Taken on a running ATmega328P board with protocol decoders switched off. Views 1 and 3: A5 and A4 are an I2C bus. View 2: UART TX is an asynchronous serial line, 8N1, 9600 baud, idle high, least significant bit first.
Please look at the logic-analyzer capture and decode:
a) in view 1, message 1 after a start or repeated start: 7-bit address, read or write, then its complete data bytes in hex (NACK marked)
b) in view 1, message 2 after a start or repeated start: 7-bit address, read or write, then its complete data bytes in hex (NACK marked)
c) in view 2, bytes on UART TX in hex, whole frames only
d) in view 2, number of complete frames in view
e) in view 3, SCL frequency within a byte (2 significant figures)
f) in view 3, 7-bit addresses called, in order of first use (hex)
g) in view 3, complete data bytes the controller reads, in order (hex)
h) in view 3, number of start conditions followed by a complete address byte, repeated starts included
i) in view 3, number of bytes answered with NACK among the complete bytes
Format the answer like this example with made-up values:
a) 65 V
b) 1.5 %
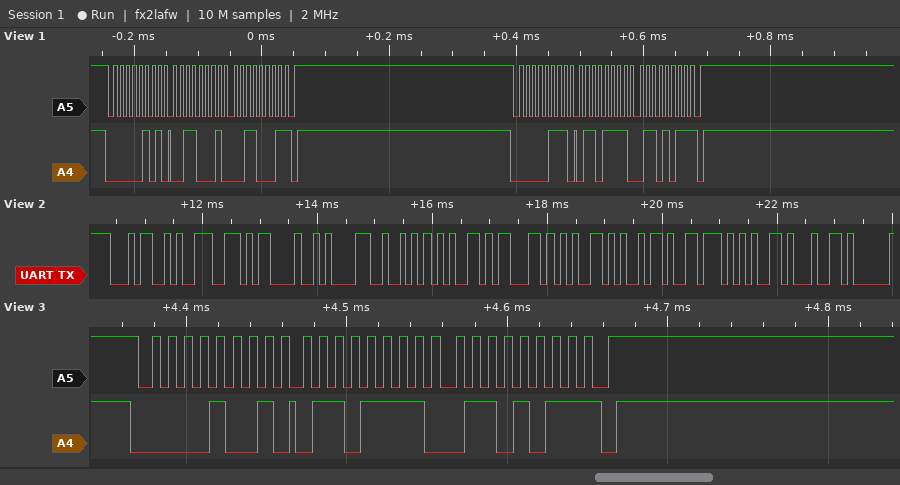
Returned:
a) 0x02 read: 31 31 NACK
b) 0x03 read: 6F 6B NACK
c) 34 39 0D 0A 52 65 63 65 69 76 65 64
d) 12
e) 100 kHz
f) 0x04
g) 6F 6B
h) 1
i) 1
